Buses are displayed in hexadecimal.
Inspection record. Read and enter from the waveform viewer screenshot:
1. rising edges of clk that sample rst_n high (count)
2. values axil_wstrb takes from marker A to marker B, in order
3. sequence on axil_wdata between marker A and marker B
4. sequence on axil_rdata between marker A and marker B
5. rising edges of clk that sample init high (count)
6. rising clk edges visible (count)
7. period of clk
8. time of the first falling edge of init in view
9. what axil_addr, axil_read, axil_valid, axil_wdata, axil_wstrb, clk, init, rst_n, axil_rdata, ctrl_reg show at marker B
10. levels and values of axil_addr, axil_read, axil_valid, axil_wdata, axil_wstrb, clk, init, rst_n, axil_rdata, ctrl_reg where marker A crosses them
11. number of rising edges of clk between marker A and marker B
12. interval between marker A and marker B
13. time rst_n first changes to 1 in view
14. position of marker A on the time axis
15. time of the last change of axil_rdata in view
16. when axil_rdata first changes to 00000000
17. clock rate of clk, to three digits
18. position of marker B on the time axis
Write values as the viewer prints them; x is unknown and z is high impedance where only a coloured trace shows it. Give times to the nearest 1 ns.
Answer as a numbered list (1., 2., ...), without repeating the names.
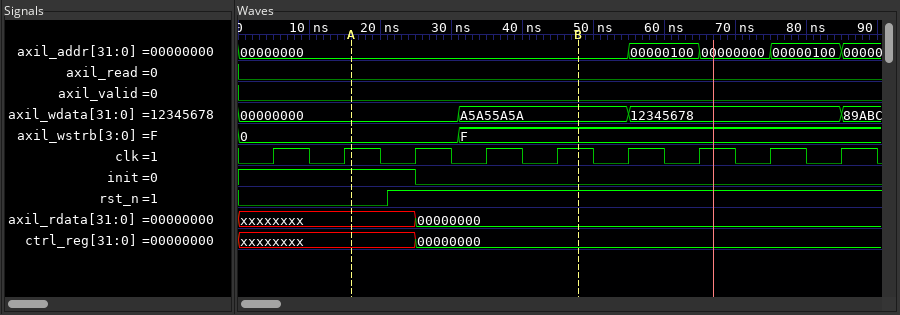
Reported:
1. 7
2. 0, F
3. 00000000, A5A55A5A
4. xxxxxxxx, 00000000
5. 3
6. 9
7. 10 ns
8. 25 ns
9. axil_addr=00000000, axil_read=0, axil_valid=0, axil_wdata=A5A55A5A, axil_wstrb=F, clk=1, init=0, rst_n=1, axil_rdata=00000000, ctrl_reg=00000000
10. axil_addr=00000000, axil_read=0, axil_valid=0, axil_wdata=00000000, axil_wstrb=0, clk=1, init=1, rst_n=0, axil_rdata=xxxxxxxx, ctrl_reg=xxxxxxxx
11. 3
12. 32 ns
13. 21 ns
14. 16 ns
15. 25 ns
16. 25 ns
17. 100 MHz
18. 48 ns
